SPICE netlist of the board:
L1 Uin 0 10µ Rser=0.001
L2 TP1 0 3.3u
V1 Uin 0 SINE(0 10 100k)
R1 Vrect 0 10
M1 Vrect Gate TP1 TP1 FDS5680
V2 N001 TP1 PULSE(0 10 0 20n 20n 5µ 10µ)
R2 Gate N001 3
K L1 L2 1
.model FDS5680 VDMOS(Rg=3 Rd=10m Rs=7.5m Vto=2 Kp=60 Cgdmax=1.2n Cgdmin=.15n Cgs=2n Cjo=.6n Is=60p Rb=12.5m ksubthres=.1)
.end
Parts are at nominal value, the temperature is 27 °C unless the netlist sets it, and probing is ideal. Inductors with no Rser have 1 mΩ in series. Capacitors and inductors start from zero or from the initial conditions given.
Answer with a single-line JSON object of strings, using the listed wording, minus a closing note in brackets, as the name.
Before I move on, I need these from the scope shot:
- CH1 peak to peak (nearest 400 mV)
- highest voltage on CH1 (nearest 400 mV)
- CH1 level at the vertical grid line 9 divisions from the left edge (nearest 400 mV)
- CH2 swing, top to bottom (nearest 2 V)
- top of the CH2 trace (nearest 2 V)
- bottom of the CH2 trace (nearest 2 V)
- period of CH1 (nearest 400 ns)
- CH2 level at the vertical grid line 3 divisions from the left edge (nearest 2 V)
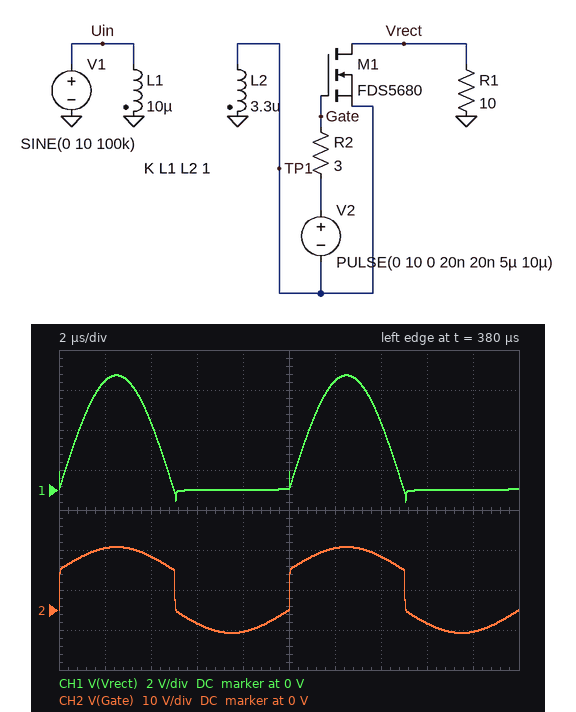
{"CH1 peak to peak": "6.4 V", "highest voltage on CH1": "5.6 V", "CH1 level at the vertical grid line 9 divisions from the left edge": "0 V", "CH2 swing, top to bottom": "22 V", "top of the CH2 trace": "16 V", "bottom of the CH2 trace": "-6 V", "period of CH1": "10.0 µs", "CH2 level at the vertical grid line 3 divisions from the left edge": "-4 V"}
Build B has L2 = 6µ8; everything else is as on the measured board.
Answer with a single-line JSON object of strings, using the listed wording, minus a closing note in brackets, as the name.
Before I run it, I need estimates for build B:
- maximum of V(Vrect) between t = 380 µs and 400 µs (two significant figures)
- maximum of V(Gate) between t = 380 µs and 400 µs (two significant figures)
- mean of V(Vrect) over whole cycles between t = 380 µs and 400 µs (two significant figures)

{"maximum of V(Vrect) between t = 380 µs and 400 µs": "8.2 V", "maximum of V(Gate) between t = 380 µs and 400 µs": "18 V", "mean of V(Vrect) over whole cycles between t = 380 µs and 400 µs": "2.6 V"}
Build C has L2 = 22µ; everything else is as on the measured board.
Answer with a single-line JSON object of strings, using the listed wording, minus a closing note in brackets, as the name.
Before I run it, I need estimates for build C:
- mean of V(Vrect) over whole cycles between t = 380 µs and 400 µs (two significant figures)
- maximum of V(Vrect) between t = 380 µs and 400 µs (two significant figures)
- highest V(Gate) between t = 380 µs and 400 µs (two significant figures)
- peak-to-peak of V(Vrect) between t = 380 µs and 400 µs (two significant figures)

{"mean of V(Vrect) over whole cycles between t = 380 µs and 400 µs": "4.7 V", "maximum of V(Vrect) between t = 380 µs and 400 µs": "15 V", "highest V(Gate) between t = 380 µs and 400 µs": "25 V", "peak-to-peak of V(Vrect) between t = 380 µs and 400 µs": "16 V"}
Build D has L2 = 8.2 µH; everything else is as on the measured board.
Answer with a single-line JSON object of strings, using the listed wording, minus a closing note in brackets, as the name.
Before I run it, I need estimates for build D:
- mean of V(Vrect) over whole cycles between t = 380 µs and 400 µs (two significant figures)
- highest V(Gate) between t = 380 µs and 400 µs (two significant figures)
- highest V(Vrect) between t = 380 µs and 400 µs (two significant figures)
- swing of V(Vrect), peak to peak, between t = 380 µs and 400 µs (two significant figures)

{"mean of V(Vrect) over whole cycles between t = 380 µs and 400 µs": "2.9 V", "highest V(Gate) between t = 380 µs and 400 µs": "19 V", "highest V(Vrect) between t = 380 µs and 400 µs": "9.0 V", "swing of V(Vrect), peak to peak, between t = 380 µs and 400 µs": "9.7 V"}
